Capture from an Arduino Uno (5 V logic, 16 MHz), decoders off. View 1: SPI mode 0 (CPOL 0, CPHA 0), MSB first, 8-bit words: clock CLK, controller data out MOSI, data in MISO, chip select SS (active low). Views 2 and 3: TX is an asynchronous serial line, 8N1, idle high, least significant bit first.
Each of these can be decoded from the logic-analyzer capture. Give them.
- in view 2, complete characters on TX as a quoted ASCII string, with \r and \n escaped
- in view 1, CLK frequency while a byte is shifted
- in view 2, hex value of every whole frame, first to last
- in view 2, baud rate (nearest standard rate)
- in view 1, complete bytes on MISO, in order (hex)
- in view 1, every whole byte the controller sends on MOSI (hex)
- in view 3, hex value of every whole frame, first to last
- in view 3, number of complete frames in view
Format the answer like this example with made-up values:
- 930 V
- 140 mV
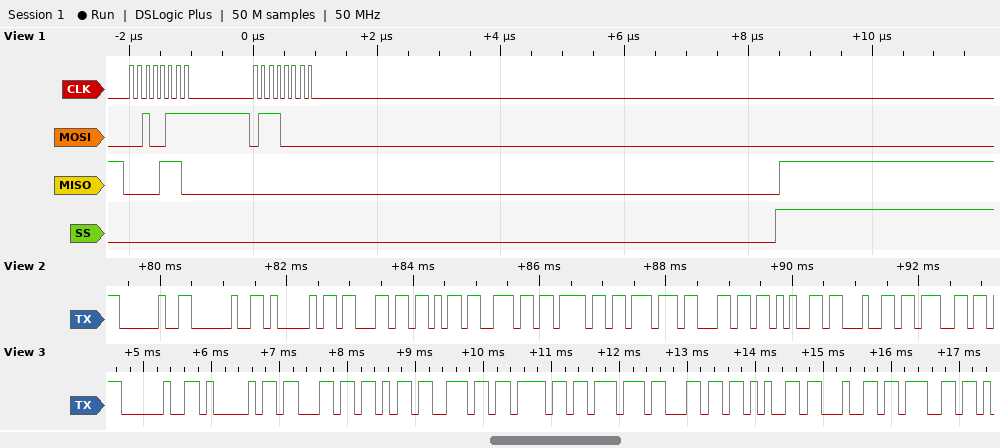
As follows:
- "  Acknowledg"
- 8 MHz
- 0x20 0x20 0x41 0x63 0x6B 0x6E 0x6F 0x77 0x6C 0x65 0x64 0x67
- 9600 baud
- 0E 00
- 27 70
- 20 41 63 6B 6E 6F 77 6C 65 64 67
- 11
